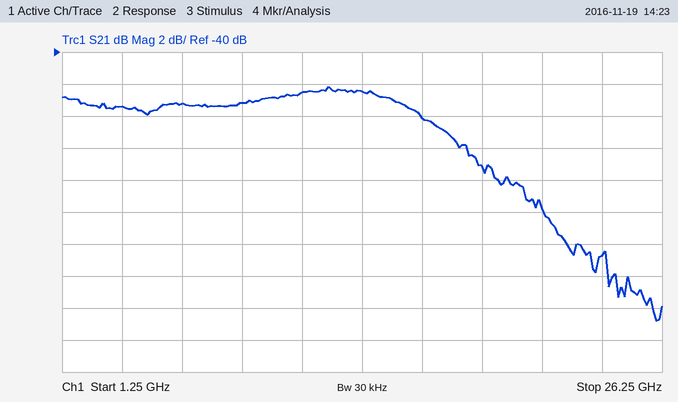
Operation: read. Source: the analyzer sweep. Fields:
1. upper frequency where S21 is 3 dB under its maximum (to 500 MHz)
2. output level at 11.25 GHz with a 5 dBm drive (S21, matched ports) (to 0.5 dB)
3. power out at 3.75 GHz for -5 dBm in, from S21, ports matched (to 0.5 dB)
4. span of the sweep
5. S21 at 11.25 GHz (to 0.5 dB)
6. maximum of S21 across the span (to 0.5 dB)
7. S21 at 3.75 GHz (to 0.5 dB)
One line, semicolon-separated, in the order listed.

17.5 GHz; -37.5 dBm; -48.5 dBm; 25 GHz; -42.5 dB; -42.0 dB; -43.5 dB
